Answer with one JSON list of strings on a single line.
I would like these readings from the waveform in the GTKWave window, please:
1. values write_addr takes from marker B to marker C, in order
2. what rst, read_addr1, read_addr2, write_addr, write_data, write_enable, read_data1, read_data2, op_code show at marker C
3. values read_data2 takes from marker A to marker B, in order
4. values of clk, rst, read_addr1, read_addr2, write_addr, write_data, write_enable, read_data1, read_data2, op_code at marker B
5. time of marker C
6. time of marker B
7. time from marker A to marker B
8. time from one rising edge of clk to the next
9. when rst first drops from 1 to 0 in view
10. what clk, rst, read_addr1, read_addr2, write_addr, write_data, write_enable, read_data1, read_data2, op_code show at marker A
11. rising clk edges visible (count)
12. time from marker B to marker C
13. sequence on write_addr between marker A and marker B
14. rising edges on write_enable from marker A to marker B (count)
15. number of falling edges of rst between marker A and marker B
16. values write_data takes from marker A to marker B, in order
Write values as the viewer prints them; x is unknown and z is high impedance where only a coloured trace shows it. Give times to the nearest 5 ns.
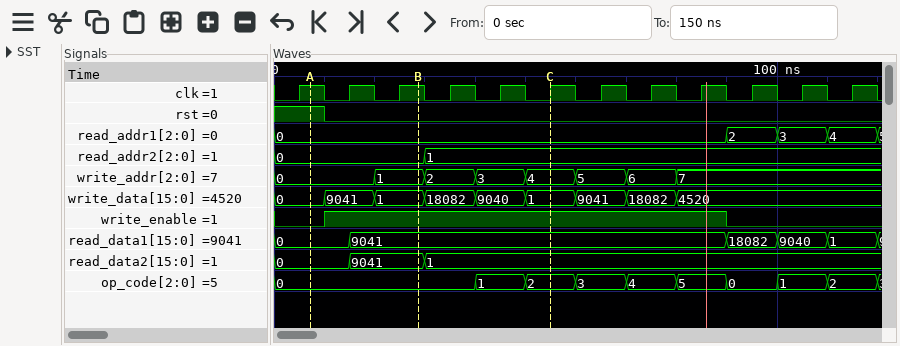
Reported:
["1, 2, 3, 4", "rst=0, read_addr1=0, read_addr2=1, write_addr=4, write_data=1, write_enable=1, read_data1=9041, read_data2=1, op_code=2", "0, 9041", "clk=1, rst=0, read_addr1=0, read_addr2=0, write_addr=1, write_data=1, write_enable=1, read_data1=9041, read_data2=9041, op_code=0", "55 ns", "30 ns", "20 ns", "10 ns", "10 ns", "clk=1, rst=1, read_addr1=0, read_addr2=0, write_addr=0, write_data=0, write_enable=0, read_data1=0, read_data2=0, op_code=0", "12", "25 ns", "0, 1", "1", "1", "0, 9041, 1"]
